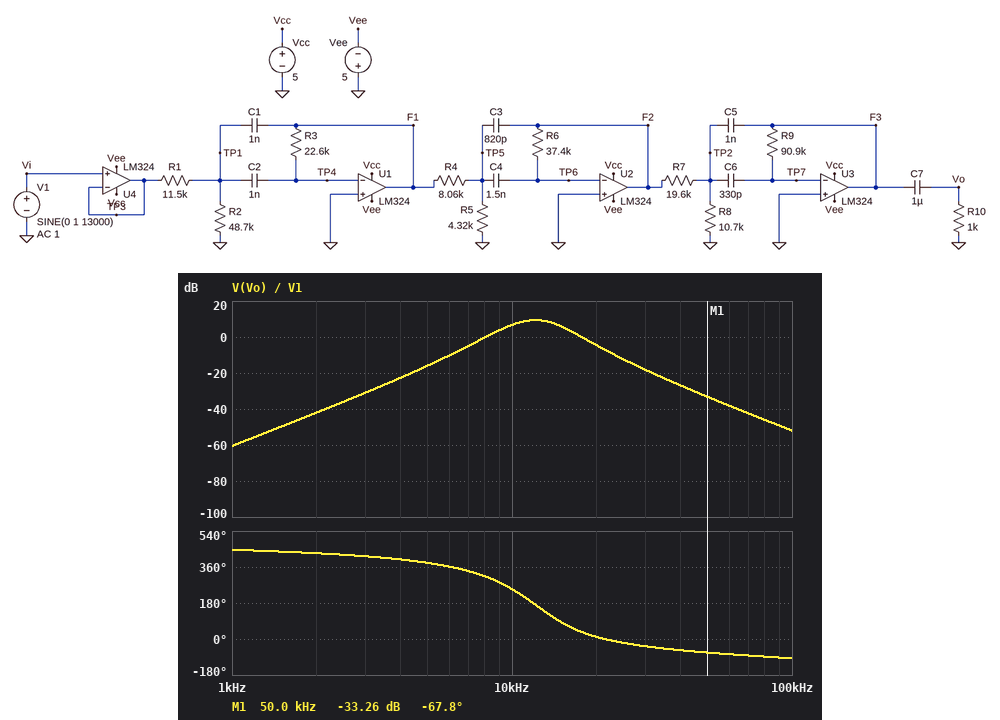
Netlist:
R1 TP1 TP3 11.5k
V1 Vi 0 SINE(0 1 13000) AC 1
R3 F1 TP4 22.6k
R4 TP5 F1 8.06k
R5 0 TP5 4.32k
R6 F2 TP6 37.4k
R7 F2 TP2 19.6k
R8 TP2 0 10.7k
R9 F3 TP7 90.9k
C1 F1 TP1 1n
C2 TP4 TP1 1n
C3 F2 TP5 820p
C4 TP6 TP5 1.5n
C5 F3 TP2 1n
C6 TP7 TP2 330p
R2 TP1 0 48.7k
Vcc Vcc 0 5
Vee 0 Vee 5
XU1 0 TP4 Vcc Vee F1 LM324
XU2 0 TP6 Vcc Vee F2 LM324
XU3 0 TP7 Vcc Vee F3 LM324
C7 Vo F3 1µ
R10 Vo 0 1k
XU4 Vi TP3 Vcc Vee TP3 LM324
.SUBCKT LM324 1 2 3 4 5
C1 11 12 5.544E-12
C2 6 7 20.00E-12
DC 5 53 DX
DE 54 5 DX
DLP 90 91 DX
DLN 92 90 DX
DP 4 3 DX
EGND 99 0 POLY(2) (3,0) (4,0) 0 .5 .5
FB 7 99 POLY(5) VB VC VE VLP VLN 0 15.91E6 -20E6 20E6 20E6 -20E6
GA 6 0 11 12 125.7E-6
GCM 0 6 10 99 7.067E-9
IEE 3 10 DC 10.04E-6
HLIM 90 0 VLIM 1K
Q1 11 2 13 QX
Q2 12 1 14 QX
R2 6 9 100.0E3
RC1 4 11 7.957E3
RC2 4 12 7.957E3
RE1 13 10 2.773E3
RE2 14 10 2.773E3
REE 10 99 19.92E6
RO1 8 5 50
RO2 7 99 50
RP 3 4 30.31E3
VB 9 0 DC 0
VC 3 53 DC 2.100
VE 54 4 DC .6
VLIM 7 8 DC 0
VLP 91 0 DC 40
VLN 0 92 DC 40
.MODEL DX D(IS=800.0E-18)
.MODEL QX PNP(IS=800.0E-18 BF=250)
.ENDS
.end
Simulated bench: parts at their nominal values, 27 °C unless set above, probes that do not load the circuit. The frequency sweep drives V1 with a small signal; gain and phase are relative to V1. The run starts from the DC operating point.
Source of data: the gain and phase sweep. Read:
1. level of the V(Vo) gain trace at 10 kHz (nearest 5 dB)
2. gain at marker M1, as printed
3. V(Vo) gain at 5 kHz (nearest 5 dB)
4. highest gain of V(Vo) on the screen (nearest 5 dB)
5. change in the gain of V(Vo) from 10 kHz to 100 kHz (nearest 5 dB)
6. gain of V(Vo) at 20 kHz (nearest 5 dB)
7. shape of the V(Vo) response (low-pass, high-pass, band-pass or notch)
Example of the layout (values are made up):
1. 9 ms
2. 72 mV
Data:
1. 5 dB
2. -33.26 dB
3. -15 dB
4. 10 dB
5. -60 dB
6. -5 dB
7. band-pass
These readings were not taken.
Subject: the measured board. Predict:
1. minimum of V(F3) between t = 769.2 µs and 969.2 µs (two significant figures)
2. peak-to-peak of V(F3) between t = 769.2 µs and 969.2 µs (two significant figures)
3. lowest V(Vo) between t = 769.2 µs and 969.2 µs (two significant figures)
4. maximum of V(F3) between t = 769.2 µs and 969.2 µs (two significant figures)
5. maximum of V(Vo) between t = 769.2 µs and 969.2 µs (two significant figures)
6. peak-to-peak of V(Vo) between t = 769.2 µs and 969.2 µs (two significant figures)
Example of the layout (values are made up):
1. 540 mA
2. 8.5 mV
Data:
1. -2.8 V
2. 5.6 V
3. -2.8 V
4. 2.8 V
5. 2.8 V
6. 5.6 V
